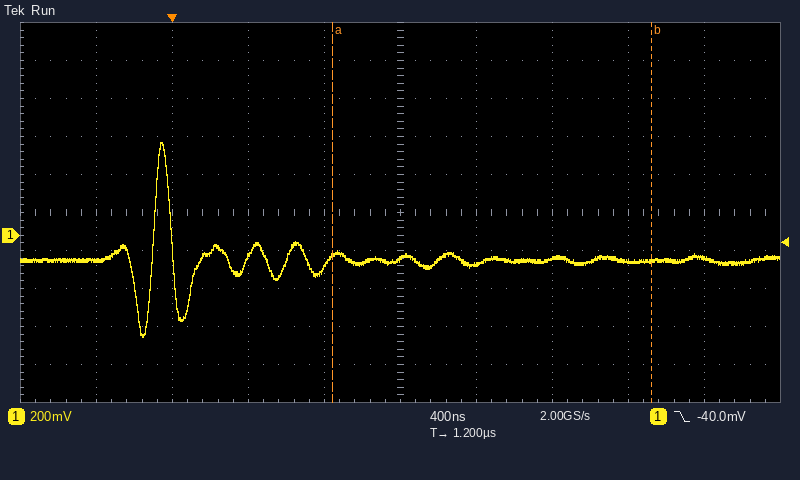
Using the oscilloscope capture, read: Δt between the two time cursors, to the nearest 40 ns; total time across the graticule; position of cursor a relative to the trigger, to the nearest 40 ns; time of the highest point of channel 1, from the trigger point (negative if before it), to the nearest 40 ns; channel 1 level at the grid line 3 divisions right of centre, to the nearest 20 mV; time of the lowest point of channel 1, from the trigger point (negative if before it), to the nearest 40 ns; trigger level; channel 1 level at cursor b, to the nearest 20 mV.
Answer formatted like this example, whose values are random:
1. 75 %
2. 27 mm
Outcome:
1. 1.68 µs
2. 4 µs
3. +840 ns
4. -40 ns
5. -140 mV
6. -160 ns
7. -40.0 mV
8. -140 mV
